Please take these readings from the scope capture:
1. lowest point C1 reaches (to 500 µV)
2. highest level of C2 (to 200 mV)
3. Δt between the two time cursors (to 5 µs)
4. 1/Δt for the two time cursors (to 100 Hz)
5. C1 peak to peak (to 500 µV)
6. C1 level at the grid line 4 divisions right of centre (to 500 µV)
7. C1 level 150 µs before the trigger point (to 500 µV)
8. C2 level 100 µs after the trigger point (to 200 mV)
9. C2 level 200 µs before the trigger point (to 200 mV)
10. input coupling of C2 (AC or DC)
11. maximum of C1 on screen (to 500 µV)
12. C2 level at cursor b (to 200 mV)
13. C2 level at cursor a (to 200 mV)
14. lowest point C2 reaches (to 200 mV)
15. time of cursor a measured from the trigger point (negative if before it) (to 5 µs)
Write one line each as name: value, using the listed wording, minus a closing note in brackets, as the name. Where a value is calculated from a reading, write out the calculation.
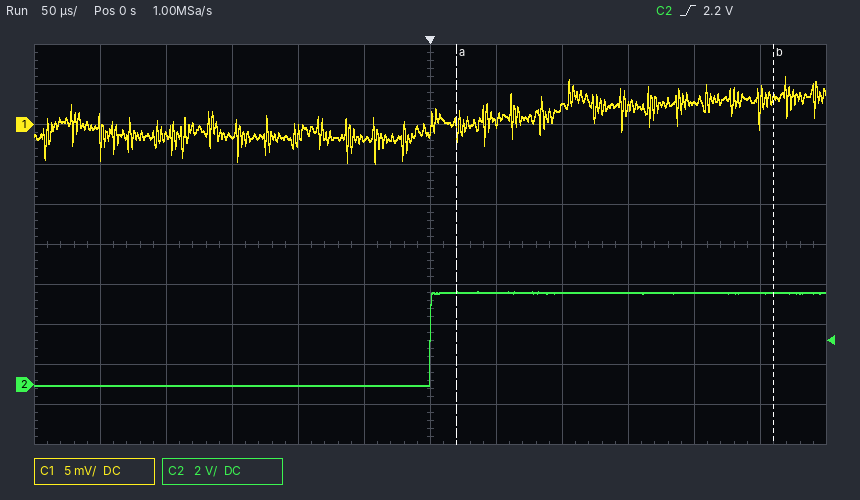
lowest point C1 reaches: -5.0 mV
highest level of C2: 4.6 V
Δt between the two time cursors: 240 µs
1/Δt for the two time cursors: 1 / 240 µs ≈ 4.2 kHz
C1 peak to peak: 6.0 mV − (-5.0 mV) = 11.0 mV
C1 level at the grid line 4 divisions right of centre: 2.5 mV
C1 level 150 µs before the trigger point: -1.5 mV
C2 level 100 µs after the trigger point: 4.6 V
C2 level 200 µs before the trigger point: 0.0 V
input coupling of C2: DC
maximum of C1 on screen: 6.0 mV
C2 level at cursor b: 4.6 V
C2 level at cursor a: 4.6 V
lowest point C2 reaches: 0.0 V
time of cursor a measured from the trigger point (negative if before it): +20 µs
